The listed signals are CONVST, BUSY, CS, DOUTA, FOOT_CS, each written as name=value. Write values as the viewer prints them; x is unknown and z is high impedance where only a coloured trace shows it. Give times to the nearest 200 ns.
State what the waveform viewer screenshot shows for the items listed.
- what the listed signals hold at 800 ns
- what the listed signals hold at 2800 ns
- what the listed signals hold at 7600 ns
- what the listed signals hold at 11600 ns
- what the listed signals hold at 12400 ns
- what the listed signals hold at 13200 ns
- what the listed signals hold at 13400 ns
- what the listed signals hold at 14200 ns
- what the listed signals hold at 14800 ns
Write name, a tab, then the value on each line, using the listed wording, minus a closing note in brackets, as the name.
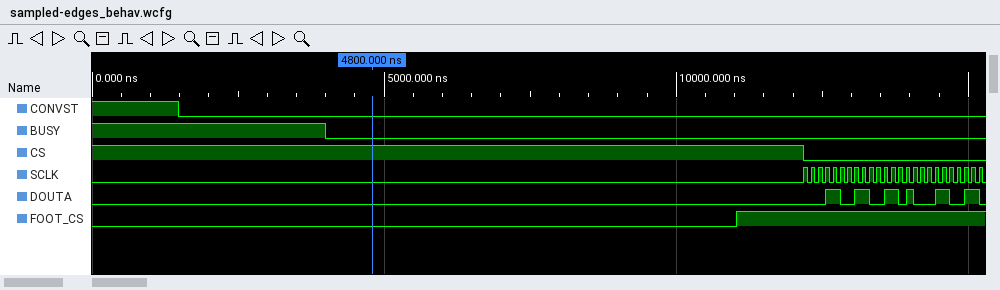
what the listed signals hold at 800 ns	CONVST=1, BUSY=1, CS=1, DOUTA=0, FOOT_CS=0
what the listed signals hold at 2800 ns	CONVST=0, BUSY=1, CS=1, DOUTA=0, FOOT_CS=0
what the listed signals hold at 7600 ns	CONVST=0, BUSY=0, CS=1, DOUTA=0, FOOT_CS=0
what the listed signals hold at 11600 ns	CONVST=0, BUSY=0, CS=1, DOUTA=0, FOOT_CS=1
what the listed signals hold at 12400 ns	CONVST=0, BUSY=0, CS=0, DOUTA=0, FOOT_CS=1
what the listed signals hold at 13200 ns	CONVST=0, BUSY=0, CS=0, DOUTA=1, FOOT_CS=1
what the listed signals hold at 13400 ns	CONVST=0, BUSY=0, CS=0, DOUTA=0, FOOT_CS=1
what the listed signals hold at 14200 ns	CONVST=0, BUSY=0, CS=0, DOUTA=0, FOOT_CS=1
what the listed signals hold at 14800 ns	CONVST=0, BUSY=0, CS=0, DOUTA=0, FOOT_CS=1
